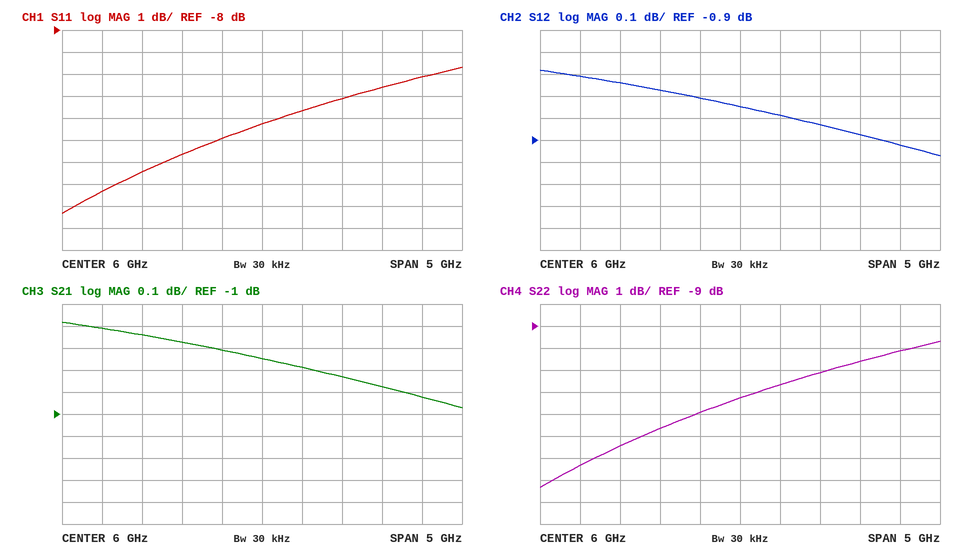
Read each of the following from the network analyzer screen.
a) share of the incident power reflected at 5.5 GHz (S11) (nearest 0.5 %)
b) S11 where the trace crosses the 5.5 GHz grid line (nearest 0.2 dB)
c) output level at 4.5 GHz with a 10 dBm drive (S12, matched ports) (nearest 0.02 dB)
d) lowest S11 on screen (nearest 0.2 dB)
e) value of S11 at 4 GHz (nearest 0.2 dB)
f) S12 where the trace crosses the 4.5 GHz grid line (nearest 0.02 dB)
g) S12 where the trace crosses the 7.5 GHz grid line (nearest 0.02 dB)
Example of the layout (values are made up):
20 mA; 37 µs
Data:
5.0 %; -13.0 dB; 9.36 dBm; -16.4 dB; -15.4 dB; -0.64 dB; -0.88 dB
